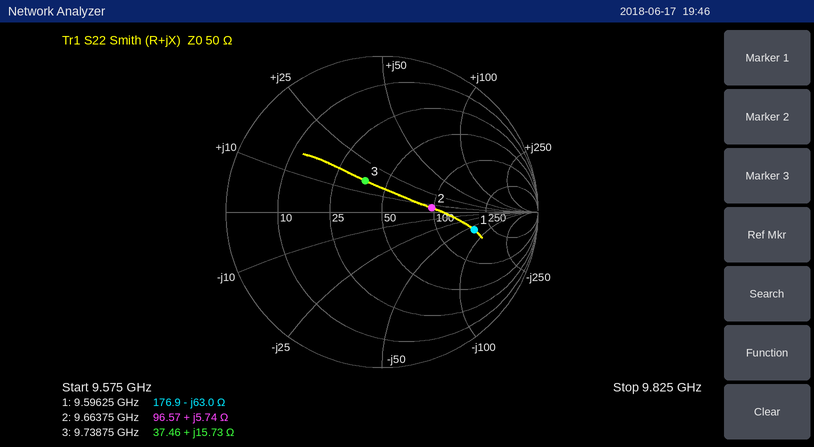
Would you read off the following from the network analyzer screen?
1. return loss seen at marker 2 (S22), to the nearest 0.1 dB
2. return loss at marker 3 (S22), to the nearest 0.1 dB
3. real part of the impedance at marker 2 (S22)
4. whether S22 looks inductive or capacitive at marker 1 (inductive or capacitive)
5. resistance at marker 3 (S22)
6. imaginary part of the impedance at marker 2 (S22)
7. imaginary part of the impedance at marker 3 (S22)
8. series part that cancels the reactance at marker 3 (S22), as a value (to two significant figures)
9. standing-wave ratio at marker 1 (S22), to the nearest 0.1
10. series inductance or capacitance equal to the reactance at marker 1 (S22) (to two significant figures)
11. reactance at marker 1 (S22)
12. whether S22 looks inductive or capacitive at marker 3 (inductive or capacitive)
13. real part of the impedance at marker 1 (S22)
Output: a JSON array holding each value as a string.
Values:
["9.9 dB", "12.9 dB", "96.57 Ω", "capacitive", "37.46 Ω", "+5.74 Ω", "+15.73 Ω", "1.0 pF", "4.0", "260 fF", "-63.0 Ω", "inductive", "176.9 Ω"]
